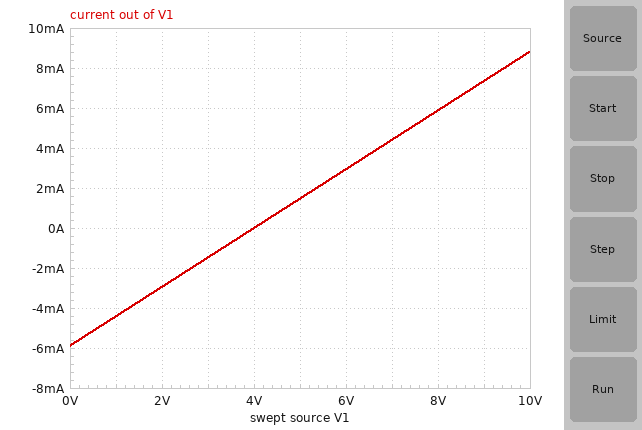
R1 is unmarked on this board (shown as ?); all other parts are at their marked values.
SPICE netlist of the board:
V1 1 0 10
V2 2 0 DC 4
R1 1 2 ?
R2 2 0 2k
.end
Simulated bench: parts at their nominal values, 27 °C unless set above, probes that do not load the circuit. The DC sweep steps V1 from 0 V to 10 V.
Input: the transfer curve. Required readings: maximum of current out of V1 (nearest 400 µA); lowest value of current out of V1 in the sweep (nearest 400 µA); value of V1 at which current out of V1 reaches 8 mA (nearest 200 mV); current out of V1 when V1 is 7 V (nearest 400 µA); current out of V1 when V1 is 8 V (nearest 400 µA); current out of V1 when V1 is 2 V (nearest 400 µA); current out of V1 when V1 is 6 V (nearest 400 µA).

8.8 mA
-6.0 mA
9.4 V
4.4 mA
6.0 mA
-2.8 mA
2.8 mA
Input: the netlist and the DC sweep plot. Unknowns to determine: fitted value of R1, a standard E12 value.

680 Ω
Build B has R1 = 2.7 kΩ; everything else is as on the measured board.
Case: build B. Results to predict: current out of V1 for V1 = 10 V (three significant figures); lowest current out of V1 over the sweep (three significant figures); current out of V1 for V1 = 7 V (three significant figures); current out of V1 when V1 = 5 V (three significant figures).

2.22 mA
-1.48 mA
1.11 mA
370 µA
